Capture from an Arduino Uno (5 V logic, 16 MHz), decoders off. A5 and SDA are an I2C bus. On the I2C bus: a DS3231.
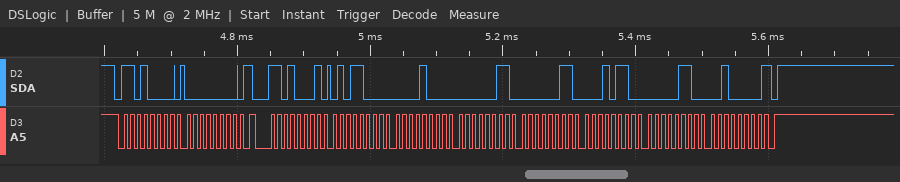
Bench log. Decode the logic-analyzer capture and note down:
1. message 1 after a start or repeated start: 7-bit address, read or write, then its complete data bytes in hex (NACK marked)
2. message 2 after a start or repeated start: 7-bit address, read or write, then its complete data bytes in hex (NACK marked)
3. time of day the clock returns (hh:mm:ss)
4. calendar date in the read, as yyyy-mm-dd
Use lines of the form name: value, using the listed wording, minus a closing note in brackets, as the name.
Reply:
message 1 after a start or repeated start: 7-bit address, read or write, then its complete data bytes in hex: 0x68 write: 00
message 2 after a start or repeated start: 7-bit address, read or write, then its complete data bytes in hex: 0x68 read: 58 08 03 03 16 06 20 NACK
time of day the clock returns: 03:08:58
calendar date in the read, as yyyy-mm-dd: 2020-06-16
